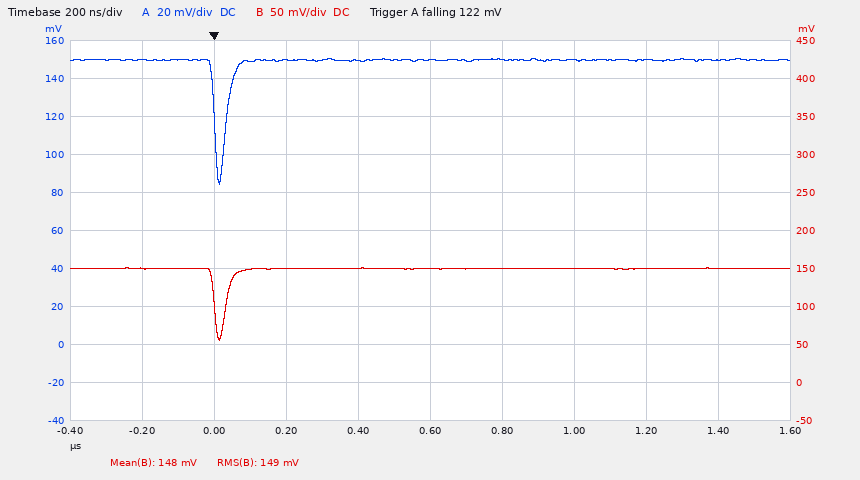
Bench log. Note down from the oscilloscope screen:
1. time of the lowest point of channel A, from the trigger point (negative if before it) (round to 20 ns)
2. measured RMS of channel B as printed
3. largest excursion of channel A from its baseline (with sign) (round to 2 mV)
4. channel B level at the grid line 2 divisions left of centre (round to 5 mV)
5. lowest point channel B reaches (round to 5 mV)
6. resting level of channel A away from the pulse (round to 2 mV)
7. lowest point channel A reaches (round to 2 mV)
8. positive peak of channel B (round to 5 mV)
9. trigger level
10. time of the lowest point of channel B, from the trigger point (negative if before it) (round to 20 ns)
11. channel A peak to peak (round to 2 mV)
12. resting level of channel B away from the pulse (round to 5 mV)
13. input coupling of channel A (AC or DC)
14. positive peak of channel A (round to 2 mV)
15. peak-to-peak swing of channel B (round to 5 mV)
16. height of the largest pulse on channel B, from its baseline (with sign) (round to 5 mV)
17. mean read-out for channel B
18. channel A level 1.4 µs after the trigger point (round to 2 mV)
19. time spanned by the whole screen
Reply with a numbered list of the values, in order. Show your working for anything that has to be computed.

1. +20 ns
2. 149 mV
3. 84 mV − (150 mV) = -66 mV
4. 150 mV
5. 55 mV
6. 150 mV
7. 84 mV
8. 150 mV
9. 122 mV
10. +20 ns
11. 150 mV − (84 mV) = 66 mV
12. 150 mV
13. DC
14. 150 mV
15. 150 mV − (55 mV) = 95 mV
16. 55 mV − (150 mV) = -95 mV
17. 148 mV
18. 150 mV
19. 2 µs
